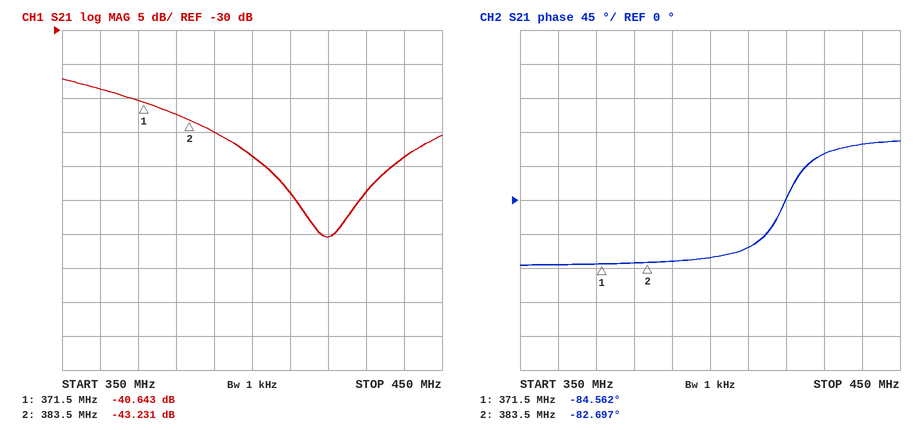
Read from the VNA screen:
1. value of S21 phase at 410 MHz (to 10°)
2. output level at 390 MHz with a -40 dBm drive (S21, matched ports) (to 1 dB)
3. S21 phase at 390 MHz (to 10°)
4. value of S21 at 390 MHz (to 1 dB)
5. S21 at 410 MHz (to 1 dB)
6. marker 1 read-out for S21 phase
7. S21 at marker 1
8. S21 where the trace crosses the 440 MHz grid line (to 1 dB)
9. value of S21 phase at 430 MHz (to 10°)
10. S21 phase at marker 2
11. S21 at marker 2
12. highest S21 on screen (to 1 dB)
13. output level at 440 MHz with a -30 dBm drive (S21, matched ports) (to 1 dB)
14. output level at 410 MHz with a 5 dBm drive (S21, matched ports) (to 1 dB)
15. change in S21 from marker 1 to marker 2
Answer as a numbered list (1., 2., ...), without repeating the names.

1. -60°
2. -85 dBm
3. -80°
4. -45 dB
5. -54 dB
6. -84.562°
7. -40.643 dB
8. -49 dB
9. 60°
10. -82.697°
11. -43.231 dB
12. -37 dB
13. -79 dBm
14. -49 dBm
15. -2.588 dB
